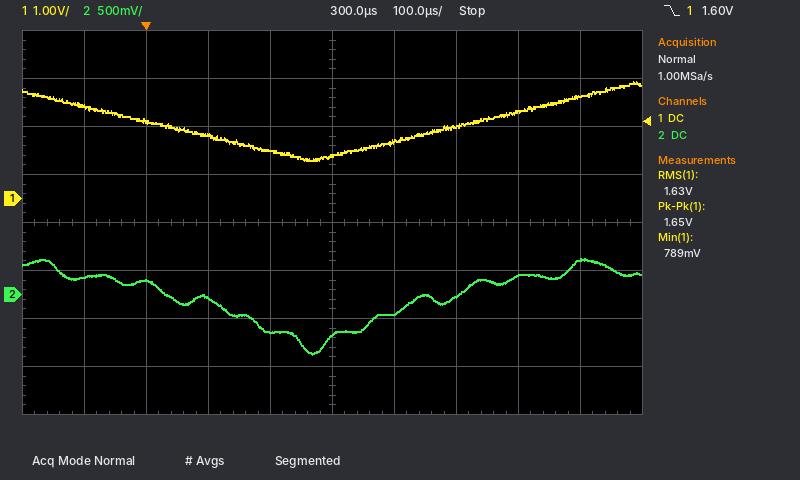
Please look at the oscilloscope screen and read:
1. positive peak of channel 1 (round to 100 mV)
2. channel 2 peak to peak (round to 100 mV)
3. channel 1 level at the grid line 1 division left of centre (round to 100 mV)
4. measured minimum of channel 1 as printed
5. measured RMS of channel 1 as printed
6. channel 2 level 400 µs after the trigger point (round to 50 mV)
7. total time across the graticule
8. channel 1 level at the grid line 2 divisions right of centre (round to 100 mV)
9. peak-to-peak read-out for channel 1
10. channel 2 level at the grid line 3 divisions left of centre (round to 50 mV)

2.4 V
1.00 V
1.0 V
789 mV
1.63 V
-200 mV
1 ms
1.5 V
1.65 V
150 mV
